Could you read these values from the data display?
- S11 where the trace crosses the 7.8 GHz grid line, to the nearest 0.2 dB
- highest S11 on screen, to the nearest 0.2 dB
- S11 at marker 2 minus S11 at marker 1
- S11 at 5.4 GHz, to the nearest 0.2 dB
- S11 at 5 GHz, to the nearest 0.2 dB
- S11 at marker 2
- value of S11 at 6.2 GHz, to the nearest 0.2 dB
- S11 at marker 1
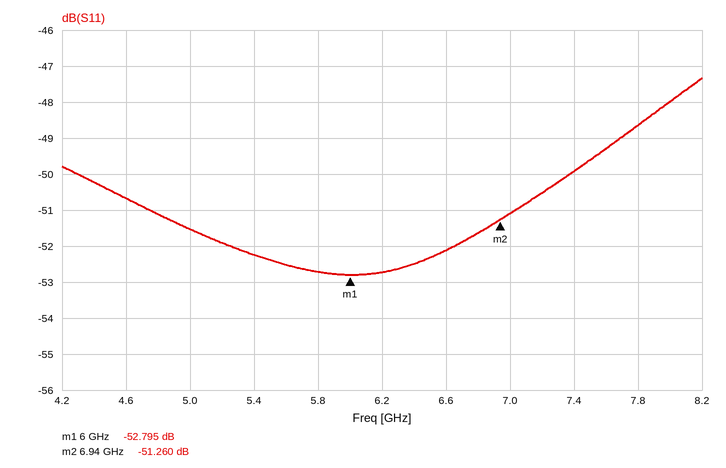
-48.6 dB
-47.4 dB
1.535 dB
-52.2 dB
-51.6 dB
-51.260 dB
-52.8 dB
-52.795 dB
